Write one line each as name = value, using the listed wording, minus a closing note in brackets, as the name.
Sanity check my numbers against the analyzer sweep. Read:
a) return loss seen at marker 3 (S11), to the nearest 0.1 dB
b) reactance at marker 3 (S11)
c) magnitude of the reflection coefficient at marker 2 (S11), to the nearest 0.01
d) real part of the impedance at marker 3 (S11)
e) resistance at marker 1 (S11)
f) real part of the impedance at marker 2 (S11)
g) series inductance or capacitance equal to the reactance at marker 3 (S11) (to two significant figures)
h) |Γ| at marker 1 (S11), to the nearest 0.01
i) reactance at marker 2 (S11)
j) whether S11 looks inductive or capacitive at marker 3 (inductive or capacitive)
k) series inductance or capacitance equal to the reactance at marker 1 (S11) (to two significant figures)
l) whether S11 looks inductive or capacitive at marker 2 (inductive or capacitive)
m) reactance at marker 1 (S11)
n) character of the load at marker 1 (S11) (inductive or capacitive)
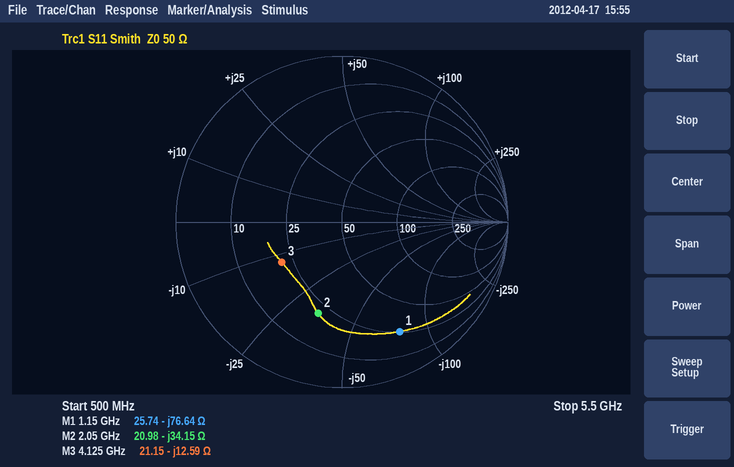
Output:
return loss seen at marker 3 (S11), to the nearest 0.1 dB = 7.2 dB
reactance at marker 3 = -12.59 Ω
magnitude of the reflection coefficient at marker 2 (S11), to the nearest 0.01 = 0.57
real part of the impedance at marker 3 = 21.15 Ω
resistance at marker 1 = 25.74 Ω
real part of the impedance at marker 2 = 20.98 Ω
series inductance or capacitance equal to the reactance at marker 3 (S11) = 3.1 pF
|Γ| at marker 1 (S11), to the nearest 0.01 = 0.75
reactance at marker 2 = -34.15 Ω
whether S11 looks inductive or capacitive at marker 3 = capacitive
series inductance or capacitance equal to the reactance at marker 1 (S11) = 1.8 pF
whether S11 looks inductive or capacitive at marker 2 = capacitive
reactance at marker 1 = -76.64 Ω
character of the load at marker 1 (S11) = capacitive
